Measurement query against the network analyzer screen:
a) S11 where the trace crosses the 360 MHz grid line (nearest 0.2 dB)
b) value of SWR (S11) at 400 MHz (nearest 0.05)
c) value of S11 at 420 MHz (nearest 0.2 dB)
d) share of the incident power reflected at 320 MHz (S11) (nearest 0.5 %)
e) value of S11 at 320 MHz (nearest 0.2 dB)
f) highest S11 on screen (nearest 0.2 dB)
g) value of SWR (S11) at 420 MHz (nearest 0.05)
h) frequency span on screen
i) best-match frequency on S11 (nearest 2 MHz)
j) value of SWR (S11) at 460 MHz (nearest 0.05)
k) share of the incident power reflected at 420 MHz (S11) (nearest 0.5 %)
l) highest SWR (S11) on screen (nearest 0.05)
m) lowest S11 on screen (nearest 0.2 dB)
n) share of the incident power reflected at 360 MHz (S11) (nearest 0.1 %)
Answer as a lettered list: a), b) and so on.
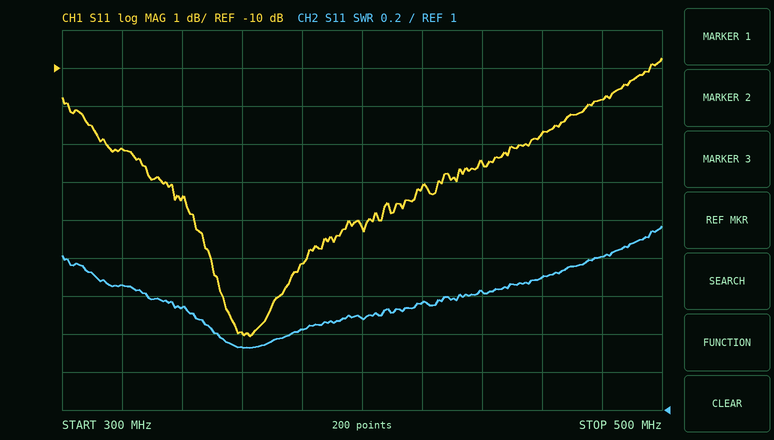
a) -17.0 dB
b) 1.50
c) -13.2 dB
d) 6.0 %
e) -12.2 dB
f) -9.8 dB
g) 1.55
h) 200 MHz
i) 362 MHz
j) 1.70
k) 5.0 %
l) 1.95
m) -17.0 dB
n) 2.0 %
